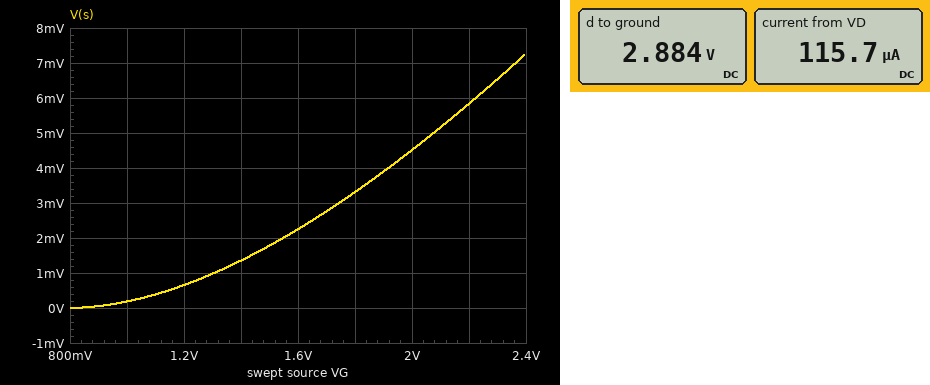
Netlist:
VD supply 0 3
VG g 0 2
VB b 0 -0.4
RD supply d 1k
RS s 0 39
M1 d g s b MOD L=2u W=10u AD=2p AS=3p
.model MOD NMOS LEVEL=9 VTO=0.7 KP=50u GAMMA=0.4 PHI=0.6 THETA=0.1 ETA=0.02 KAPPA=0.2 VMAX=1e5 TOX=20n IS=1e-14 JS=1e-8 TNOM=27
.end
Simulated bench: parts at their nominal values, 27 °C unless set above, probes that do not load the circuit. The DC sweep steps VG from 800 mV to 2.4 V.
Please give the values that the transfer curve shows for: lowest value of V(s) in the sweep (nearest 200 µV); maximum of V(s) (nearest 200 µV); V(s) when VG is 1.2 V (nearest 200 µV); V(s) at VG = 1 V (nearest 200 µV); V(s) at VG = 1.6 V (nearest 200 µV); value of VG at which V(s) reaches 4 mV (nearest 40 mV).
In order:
0 V
7.2 mV
600 µV
200 µV
2.2 mV
1.92 V
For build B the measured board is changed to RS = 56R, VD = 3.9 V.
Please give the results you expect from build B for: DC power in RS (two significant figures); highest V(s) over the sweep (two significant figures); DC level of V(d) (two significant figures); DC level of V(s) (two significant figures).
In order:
750 nW
10 mV
3.8 V
6.5 mV
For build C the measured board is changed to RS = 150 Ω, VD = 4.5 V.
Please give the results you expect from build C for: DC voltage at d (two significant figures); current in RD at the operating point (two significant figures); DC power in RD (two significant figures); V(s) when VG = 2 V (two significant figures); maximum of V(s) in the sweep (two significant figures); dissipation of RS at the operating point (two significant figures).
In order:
4.4 V
110 µA
13 µW
17 mV
27 mV
1.9 µW
